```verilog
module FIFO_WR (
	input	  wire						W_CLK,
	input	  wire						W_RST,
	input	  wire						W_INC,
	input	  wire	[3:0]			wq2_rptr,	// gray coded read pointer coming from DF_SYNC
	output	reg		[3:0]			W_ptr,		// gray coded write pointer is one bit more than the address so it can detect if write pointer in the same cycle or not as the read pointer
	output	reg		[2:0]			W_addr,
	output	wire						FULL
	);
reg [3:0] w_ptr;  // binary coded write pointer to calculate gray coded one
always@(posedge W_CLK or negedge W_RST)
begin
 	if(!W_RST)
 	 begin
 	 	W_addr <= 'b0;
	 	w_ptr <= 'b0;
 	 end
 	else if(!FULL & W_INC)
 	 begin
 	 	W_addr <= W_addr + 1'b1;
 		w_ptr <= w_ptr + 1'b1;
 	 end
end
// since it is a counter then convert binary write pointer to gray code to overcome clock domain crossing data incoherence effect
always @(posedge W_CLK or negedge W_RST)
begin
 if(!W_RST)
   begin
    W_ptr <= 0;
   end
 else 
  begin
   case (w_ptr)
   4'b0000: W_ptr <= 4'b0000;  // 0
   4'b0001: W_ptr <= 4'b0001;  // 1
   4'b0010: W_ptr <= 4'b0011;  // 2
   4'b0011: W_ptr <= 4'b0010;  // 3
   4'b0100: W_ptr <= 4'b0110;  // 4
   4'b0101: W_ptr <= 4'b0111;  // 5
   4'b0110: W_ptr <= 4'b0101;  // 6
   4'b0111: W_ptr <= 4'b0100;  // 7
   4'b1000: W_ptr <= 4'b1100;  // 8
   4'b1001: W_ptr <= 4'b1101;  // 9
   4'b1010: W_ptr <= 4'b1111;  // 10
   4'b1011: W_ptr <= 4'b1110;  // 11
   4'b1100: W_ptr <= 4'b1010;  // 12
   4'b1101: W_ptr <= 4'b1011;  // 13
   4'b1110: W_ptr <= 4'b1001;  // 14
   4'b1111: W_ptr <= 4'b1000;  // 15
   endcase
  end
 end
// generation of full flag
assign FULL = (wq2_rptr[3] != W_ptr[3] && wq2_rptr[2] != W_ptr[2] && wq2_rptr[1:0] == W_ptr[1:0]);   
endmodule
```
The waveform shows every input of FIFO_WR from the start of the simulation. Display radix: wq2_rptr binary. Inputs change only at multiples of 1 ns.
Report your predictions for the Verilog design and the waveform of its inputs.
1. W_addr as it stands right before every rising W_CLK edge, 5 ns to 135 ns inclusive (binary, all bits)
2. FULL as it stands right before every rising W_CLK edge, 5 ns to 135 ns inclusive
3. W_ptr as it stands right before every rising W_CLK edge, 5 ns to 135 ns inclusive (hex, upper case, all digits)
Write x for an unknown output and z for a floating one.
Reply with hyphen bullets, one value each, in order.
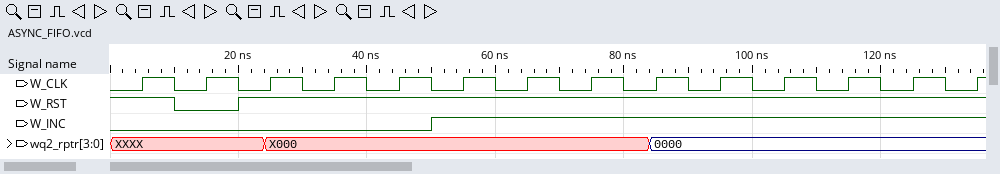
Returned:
- x, 000, 000, 000, 000, 000, 001, 010, 011, 100, 101, 110, 111, 000
- x x 0 0 0 0 0 0 0 0 0 0 0 0
- x, 0, 0, 0, 0, 0, 0, 1, 3, 2, 6, 7, 5, 4
